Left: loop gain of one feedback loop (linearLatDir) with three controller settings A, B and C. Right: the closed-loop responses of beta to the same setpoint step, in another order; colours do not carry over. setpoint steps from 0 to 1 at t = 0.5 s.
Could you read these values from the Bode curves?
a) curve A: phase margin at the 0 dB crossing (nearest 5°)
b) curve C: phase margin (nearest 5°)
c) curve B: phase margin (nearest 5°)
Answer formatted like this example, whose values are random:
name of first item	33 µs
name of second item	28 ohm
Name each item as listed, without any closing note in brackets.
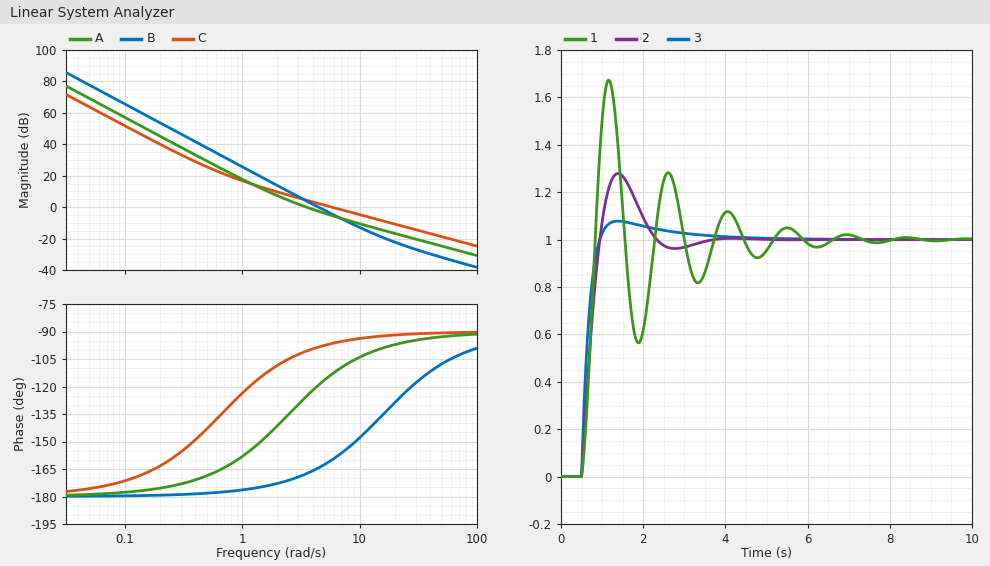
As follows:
curve A: phase margin at the 0 dB crossing	55°
curve C: phase margin	85°
curve B: phase margin	15°
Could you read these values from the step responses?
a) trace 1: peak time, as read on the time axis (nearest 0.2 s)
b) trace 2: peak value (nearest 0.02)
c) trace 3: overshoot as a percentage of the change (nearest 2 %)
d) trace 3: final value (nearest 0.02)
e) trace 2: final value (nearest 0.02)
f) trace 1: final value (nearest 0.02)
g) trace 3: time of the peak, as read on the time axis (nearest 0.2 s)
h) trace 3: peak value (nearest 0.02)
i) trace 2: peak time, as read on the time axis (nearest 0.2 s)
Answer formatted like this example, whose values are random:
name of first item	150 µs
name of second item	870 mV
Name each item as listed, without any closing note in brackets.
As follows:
trace 1: peak time, as read on the time axis	1.2 s
trace 2: peak value	1.28
trace 3: overshoot as a percentage of the change	8 %
trace 3: final value	1.00
trace 2: final value	1.00
trace 1: final value	1.00
trace 3: time of the peak, as read on the time axis	1.4 s
trace 3: peak value	1.08
trace 2: peak time, as read on the time axis	1.4 s
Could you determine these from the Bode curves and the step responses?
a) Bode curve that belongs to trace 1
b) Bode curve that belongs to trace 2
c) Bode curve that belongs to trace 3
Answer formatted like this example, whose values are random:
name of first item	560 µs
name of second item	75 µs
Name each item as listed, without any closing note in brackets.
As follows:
Bode curve that belongs to trace 1	B
Bode curve that belongs to trace 2	A
Bode curve that belongs to trace 3	C
